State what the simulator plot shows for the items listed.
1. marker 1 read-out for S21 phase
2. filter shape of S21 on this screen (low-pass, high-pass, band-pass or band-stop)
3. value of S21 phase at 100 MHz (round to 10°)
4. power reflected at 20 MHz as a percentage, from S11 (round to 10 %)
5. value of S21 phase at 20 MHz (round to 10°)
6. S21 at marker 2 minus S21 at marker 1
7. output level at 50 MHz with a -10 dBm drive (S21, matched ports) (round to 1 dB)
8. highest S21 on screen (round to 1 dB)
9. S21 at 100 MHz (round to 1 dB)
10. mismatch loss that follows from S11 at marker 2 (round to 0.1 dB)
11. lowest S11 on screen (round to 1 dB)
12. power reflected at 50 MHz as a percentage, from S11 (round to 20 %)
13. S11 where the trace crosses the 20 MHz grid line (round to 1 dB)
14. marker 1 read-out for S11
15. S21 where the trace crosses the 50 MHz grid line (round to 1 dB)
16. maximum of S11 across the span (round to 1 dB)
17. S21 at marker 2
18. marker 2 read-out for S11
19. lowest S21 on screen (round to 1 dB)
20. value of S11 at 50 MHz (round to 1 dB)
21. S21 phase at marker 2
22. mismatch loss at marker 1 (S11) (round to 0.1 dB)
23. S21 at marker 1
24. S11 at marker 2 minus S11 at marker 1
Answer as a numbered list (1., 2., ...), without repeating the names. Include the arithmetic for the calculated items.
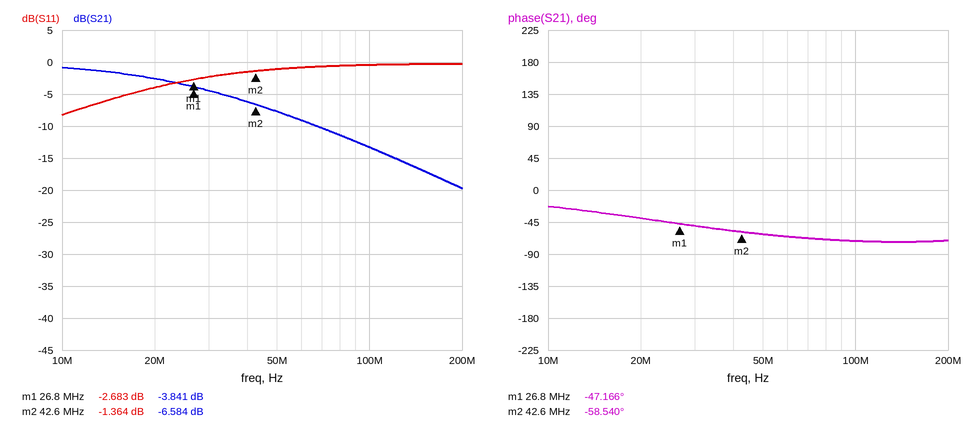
1. -47.166°
2. low-pass
3. -70°
4. 10^(-4/10) ≈ 40 %
5. -40°
6. -6.584 − (-3.841) = -2.743 dB
7. -10 dBm + (-8 dB) = -18 dBm
8. -1 dB
9. -13 dB
10. −10 log10(1 − 10^(-1.364/10)) ≈ 5.7 dB
11. -8 dB
12. 10^(-1/10) ≈ 79.4 %, so 80 % to the nearest 20 %
13. -4 dB
14. -2.683 dB
15. -8 dB
16. 0 dB
17. -6.584 dB
18. -1.364 dB
19. -20 dB
20. -1 dB
21. -58.540°
22. −10 log10(1 − 10^(-2.683/10)) ≈ 3.4 dB
23. -3.841 dB
24. -1.364 − (-2.683) = 1.319 dB
